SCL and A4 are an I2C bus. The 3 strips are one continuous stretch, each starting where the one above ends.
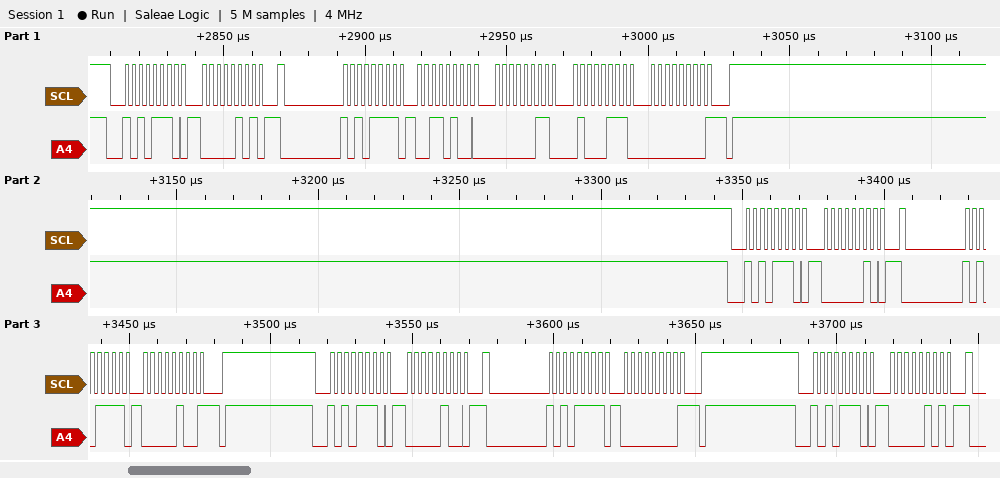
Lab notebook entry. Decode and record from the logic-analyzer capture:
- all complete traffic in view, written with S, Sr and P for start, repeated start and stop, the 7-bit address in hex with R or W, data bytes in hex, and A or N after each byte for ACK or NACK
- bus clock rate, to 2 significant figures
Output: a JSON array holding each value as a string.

["S 57W A 05 A Sr 57R A 34 A 03 A 47 A 00 N P S 57W A 02 A Sr 57R A 04 N P S 57W A 04 A Sr 57R A 00 N P S 57W A 05 A", "400 kHz"]
